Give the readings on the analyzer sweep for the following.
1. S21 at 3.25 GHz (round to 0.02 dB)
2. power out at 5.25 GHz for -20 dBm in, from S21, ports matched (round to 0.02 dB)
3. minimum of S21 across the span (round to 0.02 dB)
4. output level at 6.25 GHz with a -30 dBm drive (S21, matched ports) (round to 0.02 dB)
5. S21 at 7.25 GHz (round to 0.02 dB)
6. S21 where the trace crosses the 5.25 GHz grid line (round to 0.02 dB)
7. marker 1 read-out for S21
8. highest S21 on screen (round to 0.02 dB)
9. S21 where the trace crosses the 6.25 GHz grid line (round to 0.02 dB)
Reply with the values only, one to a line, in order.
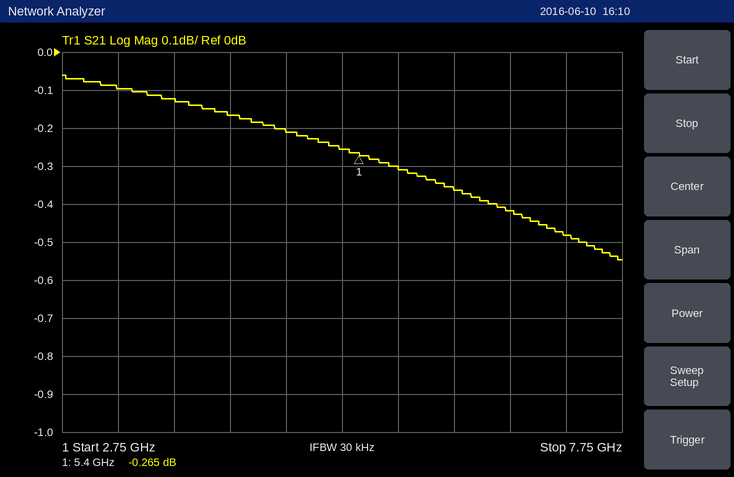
-0.10 dB
-20.26 dBm
-0.54 dB
-30.36 dBm
-0.48 dB
-0.26 dB
-0.265 dB
-0.06 dB
-0.36 dB
